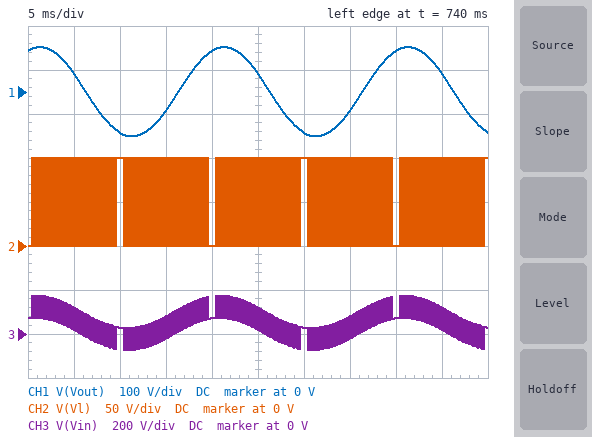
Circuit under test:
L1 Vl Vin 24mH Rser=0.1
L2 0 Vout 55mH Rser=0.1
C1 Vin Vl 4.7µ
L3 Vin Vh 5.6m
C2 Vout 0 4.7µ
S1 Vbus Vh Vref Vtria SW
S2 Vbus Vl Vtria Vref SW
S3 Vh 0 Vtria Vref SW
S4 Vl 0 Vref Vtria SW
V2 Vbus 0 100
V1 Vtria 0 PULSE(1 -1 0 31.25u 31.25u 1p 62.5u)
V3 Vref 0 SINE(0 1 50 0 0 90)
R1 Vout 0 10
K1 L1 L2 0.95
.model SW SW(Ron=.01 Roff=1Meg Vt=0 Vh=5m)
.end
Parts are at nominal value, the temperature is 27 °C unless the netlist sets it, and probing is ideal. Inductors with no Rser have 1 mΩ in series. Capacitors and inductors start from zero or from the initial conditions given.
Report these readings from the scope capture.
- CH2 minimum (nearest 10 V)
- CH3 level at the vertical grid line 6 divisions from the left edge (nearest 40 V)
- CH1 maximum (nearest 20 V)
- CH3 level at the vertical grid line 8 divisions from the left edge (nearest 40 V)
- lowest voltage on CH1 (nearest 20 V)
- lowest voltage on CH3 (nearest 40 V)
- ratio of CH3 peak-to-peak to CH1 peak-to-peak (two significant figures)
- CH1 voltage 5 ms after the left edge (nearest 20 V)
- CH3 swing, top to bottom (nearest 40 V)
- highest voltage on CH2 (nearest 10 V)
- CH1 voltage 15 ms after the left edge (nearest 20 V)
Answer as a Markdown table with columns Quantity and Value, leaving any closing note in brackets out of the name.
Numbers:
| Quantity | Value |
|---|---|
| CH2 minimum | 0 V |
| CH3 level at the vertical grid line 6 divisions from the left edge | 40 V |
| CH1 maximum | 100 V |
| CH3 level at the vertical grid line 8 divisions from the left edge | 80 V |
| lowest voltage on CH1 | -100 V |
| lowest voltage on CH3 | -80 V |
| ratio of CH3 peak-to-peak to CH1 peak-to-peak | 1.2 |
| CH1 voltage 5 ms after the left edge | 40 V |
| CH3 swing, top to bottom | 240 V |
| highest voltage on CH2 | 100 V |
| CH1 voltage 15 ms after the left edge | -40 V |
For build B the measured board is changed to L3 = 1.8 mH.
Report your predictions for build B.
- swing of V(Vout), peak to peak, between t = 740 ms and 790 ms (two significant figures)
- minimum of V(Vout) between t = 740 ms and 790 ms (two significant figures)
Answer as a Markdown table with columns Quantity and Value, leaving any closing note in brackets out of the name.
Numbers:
| Quantity | Value |
|---|---|
| swing of V(Vout), peak to peak, between t = 740 ms and 790 ms | 250 V |
| minimum of V(Vout) between t = 740 ms and 790 ms | -120 V |
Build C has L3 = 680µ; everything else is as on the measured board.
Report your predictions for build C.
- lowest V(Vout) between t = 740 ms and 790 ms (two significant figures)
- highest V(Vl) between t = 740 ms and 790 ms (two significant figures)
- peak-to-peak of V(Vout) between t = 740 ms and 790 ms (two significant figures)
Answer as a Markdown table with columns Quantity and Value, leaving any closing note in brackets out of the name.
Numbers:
| Quantity | Value |
|---|---|
| lowest V(Vout) between t = 740 ms and 790 ms | -130 V |
| highest V(Vl) between t = 740 ms and 790 ms | 100 V |
| peak-to-peak of V(Vout) between t = 740 ms and 790 ms | 260 V |
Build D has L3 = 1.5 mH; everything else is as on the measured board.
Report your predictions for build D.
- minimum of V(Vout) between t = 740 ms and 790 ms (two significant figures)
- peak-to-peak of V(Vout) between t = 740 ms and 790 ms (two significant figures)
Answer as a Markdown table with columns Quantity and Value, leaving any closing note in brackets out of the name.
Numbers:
| Quantity | Value |
|---|---|
| minimum of V(Vout) between t = 740 ms and 790 ms | -130 V |
| peak-to-peak of V(Vout) between t = 740 ms and 790 ms | 250 V |
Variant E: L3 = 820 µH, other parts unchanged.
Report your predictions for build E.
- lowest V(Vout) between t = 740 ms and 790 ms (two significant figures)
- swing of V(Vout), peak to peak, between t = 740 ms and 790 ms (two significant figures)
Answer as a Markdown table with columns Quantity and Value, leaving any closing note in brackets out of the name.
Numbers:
| Quantity | Value |
|---|---|
| lowest V(Vout) between t = 740 ms and 790 ms | -130 V |
| swing of V(Vout), peak to peak, between t = 740 ms and 790 ms | 260 V |
